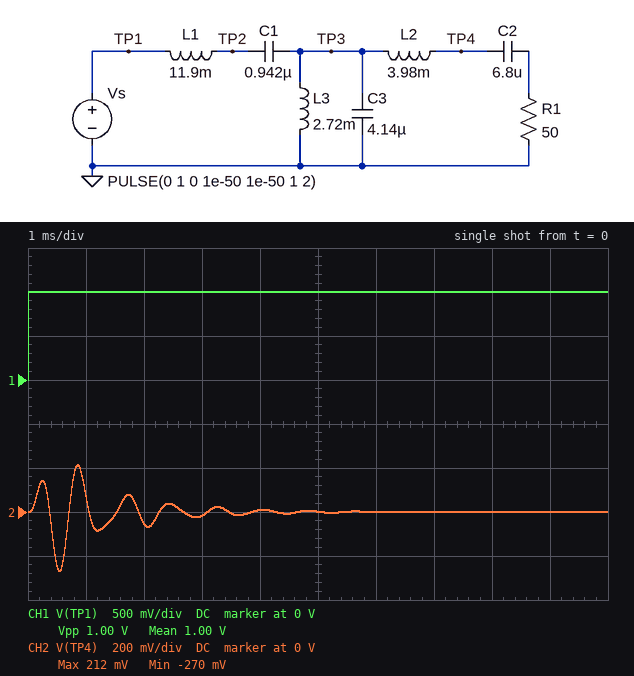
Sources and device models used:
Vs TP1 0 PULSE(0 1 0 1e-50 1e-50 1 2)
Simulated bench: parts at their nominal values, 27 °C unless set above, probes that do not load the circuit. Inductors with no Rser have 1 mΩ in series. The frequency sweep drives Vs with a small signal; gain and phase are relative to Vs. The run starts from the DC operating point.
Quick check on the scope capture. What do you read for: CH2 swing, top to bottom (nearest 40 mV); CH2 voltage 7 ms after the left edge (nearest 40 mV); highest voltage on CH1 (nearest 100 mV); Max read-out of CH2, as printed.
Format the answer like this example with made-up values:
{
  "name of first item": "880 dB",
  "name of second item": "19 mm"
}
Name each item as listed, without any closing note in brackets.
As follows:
{
  "CH2 swing, top to bottom": "480 mV",
  "CH2 voltage 7 ms after the left edge": "0 V",
  "highest voltage on CH1": "1.0 V",
  "Max read-out of CH2, as printed": "212 mV"
}
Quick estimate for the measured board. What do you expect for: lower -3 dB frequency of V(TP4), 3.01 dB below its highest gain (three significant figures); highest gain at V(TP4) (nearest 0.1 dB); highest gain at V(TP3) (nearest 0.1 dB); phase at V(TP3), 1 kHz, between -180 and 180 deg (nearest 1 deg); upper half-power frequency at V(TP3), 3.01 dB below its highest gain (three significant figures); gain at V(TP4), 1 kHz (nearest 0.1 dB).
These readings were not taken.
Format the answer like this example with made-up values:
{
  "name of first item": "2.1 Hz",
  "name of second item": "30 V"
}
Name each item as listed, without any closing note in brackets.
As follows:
{
  "lower -3 dB frequency of V(TP4), 3.01 dB below its highest gain": "1.18 kHz",
  "highest gain at V(TP4)": "2.6 dB",
  "highest gain at V(TP3)": "2.4 dB",
  "phase at V(TP3), 1 kHz, between -180 and 180 deg": "138 deg",
  "upper half-power frequency at V(TP3), 3.01 dB below its highest gain": "2.14 kHz",
  "gain at V(TP4), 1 kHz": "-8.2 dB"
}
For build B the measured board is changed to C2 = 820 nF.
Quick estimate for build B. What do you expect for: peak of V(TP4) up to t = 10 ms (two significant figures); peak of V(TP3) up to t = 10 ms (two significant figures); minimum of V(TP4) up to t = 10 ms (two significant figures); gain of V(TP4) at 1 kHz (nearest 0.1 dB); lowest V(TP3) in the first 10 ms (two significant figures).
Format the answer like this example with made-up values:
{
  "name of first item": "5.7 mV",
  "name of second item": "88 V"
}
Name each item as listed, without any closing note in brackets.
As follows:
{
  "peak of V(TP4) up to t = 10 ms": "460 mV",
  "peak of V(TP3) up to t = 10 ms": "350 mV",
  "minimum of V(TP4) up to t = 10 ms": "-440 mV",
  "gain of V(TP4) at 1 kHz": "-2.7 dB",
  "lowest V(TP3) in the first 10 ms": "-340 mV"
}
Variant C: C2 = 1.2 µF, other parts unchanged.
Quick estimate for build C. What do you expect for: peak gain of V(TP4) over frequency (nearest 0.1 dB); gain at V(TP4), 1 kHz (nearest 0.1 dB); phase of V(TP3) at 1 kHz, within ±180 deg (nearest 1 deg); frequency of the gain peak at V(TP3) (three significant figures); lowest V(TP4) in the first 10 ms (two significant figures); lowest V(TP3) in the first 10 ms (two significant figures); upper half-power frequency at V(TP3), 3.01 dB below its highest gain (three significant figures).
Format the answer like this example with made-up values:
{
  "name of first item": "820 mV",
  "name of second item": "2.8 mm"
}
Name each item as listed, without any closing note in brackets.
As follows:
{
  "peak gain of V(TP4) over frequency": "11.9 dB",
  "gain at V(TP4), 1 kHz": "-1.3 dB",
  "phase of V(TP3) at 1 kHz, within ±180 deg": "166 deg",
  "frequency of the gain peak at V(TP3)": "1.12 kHz",
  "lowest V(TP4) in the first 10 ms": "-420 mV",
  "lowest V(TP3) in the first 10 ms": "-310 mV",
  "upper half-power frequency at V(TP3), 3.01 dB below its highest gain": "1.16 kHz"
}
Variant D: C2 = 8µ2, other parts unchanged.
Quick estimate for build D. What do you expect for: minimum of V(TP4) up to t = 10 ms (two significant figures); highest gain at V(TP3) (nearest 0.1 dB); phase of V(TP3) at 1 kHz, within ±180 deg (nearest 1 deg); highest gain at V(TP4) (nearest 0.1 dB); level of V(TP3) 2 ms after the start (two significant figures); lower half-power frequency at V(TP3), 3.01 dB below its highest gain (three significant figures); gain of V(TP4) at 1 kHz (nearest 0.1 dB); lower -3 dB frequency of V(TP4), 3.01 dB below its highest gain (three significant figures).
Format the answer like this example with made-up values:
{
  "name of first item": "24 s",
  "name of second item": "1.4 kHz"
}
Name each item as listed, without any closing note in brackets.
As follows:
{
  "minimum of V(TP4) up to t = 10 ms": "-260 mV",
  "highest gain at V(TP3)": "2.8 dB",
  "phase of V(TP3) at 1 kHz, within ±180 deg": "141 deg",
  "highest gain at V(TP4)": "2.7 dB",
  "level of V(TP3) 2 ms after the start": "-78 mV",
  "lower half-power frequency at V(TP3), 3.01 dB below its highest gain": "1.19 kHz",
  "gain of V(TP4) at 1 kHz": "-8.8 dB",
  "lower -3 dB frequency of V(TP4), 3.01 dB below its highest gain": "1.18 kHz"
}
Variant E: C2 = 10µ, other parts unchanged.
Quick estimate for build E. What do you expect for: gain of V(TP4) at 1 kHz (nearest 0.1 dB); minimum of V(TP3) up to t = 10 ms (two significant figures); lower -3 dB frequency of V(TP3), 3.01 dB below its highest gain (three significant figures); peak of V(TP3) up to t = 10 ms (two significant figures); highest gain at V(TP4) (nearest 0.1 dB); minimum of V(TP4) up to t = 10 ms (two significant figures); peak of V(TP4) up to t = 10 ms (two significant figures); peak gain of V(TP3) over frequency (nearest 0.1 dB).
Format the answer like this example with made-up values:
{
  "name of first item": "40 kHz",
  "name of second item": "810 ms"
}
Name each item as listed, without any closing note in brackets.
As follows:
{
  "gain of V(TP4) at 1 kHz": "-9.3 dB",
  "minimum of V(TP3) up to t = 10 ms": "-290 mV",
  "lower -3 dB frequency of V(TP3), 3.01 dB below its highest gain": "1.19 kHz",
  "peak of V(TP3) up to t = 10 ms": "240 mV",
  "highest gain at V(TP4)": "2.8 dB",
  "minimum of V(TP4) up to t = 10 ms": "-260 mV",
  "peak of V(TP4) up to t = 10 ms": "200 mV",
  "peak gain of V(TP3) over frequency": "3.2 dB"
}
